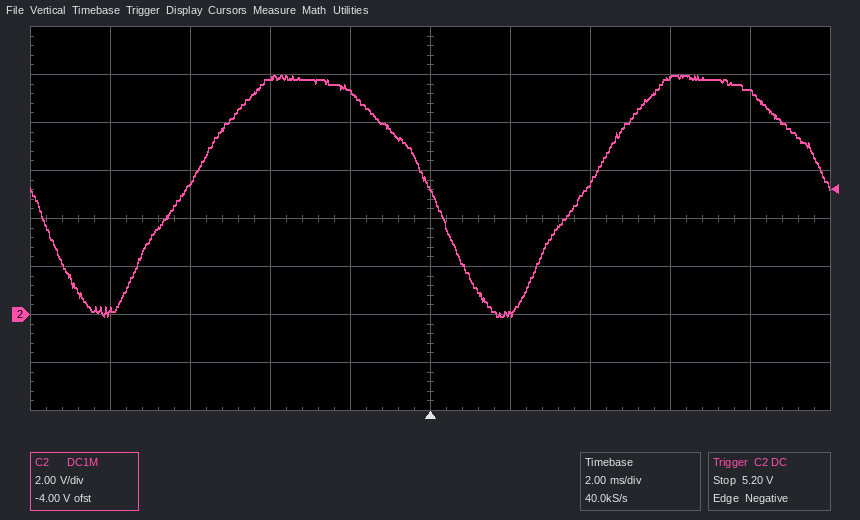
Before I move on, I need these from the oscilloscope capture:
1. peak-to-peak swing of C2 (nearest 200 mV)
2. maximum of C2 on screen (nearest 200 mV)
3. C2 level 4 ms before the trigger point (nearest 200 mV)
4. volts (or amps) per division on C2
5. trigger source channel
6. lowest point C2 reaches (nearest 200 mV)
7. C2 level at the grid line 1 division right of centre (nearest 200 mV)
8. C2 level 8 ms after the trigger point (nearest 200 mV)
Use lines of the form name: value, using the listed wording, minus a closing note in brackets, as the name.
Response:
peak-to-peak swing of C2: 10.0 V
maximum of C2 on screen: 10.0 V
C2 level 4 ms before the trigger point: 9.8 V
volts (or amps) per division on C2: 2 V
trigger source channel: C2
lowest point C2 reaches: 0.0 V
C2 level at the grid line 1 division right of centre: 0.0 V
C2 level 8 ms after the trigger point: 9.2 V
